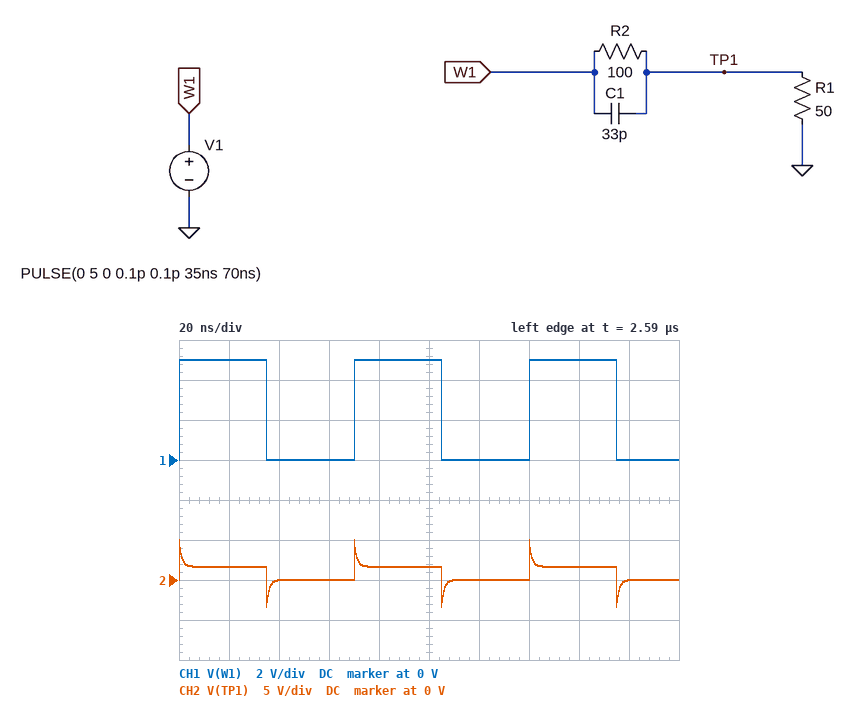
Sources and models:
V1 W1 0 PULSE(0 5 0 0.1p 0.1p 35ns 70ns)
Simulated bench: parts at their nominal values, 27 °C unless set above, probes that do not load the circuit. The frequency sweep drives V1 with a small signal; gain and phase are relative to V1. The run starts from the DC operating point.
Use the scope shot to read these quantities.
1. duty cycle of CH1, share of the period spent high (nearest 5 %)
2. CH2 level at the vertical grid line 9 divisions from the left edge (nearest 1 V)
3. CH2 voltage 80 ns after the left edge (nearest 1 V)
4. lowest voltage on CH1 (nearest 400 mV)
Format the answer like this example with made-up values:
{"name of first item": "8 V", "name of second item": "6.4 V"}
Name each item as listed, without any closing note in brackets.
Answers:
{"duty cycle of CH1, share of the period spent high": "50 %", "CH2 level at the vertical grid line 9 divisions from the left edge": "0 V", "CH2 voltage 80 ns after the left edge": "2 V", "lowest voltage on CH1": "0 V"}
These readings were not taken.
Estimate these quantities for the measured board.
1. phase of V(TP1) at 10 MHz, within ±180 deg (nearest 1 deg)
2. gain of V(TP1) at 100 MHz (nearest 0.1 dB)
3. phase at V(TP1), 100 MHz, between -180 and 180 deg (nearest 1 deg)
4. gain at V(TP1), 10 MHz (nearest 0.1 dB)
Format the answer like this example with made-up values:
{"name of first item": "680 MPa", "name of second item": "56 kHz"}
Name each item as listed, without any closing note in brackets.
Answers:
{"phase of V(TP1) at 10 MHz, within ±180 deg": "8 deg", "gain of V(TP1) at 100 MHz": "-4.0 dB", "phase at V(TP1), 100 MHz, between -180 and 180 deg": "30 deg", "gain at V(TP1), 10 MHz": "-9.4 dB"}
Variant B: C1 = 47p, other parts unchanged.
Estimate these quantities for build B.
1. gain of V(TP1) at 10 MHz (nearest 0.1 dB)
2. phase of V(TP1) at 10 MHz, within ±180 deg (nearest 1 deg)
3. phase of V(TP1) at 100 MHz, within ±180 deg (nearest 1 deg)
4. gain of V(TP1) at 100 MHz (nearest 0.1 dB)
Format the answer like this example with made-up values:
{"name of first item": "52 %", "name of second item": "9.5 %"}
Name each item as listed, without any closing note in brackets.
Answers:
{"gain of V(TP1) at 10 MHz": "-9.2 dB", "phase of V(TP1) at 10 MHz, within ±180 deg": "11 deg", "phase of V(TP1) at 100 MHz, within ±180 deg": "27 deg", "gain of V(TP1) at 100 MHz": "-2.6 dB"}
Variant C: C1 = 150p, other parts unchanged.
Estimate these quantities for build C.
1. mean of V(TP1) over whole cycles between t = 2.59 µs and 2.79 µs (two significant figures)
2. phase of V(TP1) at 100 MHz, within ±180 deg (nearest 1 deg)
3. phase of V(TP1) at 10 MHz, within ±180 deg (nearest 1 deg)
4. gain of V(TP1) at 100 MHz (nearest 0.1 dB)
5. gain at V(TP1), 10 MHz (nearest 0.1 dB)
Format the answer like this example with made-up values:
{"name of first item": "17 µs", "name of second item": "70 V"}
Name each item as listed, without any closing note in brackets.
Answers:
{"mean of V(TP1) over whole cycles between t = 2.59 µs and 2.79 µs": "830 mV", "phase of V(TP1) at 100 MHz, within ±180 deg": "12 deg", "phase of V(TP1) at 10 MHz, within ±180 deg": "26 deg", "gain of V(TP1) at 100 MHz": "-0.4 dB", "gain at V(TP1), 10 MHz": "-7.2 dB"}
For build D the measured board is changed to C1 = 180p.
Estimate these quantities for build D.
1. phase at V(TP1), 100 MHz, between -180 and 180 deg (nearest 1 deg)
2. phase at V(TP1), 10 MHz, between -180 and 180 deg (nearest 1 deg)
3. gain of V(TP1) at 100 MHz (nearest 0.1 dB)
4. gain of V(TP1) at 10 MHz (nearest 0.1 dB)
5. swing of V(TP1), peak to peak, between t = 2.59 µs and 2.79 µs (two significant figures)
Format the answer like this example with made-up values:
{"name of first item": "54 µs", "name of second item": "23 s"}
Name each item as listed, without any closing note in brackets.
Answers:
{"phase at V(TP1), 100 MHz, between -180 and 180 deg": "10 deg", "phase at V(TP1), 10 MHz, between -180 and 180 deg": "28 deg", "gain of V(TP1) at 100 MHz": "-0.3 dB", "gain of V(TP1) at 10 MHz": "-6.5 dB", "swing of V(TP1), peak to peak, between t = 2.59 µs and 2.79 µs": "8.3 V"}
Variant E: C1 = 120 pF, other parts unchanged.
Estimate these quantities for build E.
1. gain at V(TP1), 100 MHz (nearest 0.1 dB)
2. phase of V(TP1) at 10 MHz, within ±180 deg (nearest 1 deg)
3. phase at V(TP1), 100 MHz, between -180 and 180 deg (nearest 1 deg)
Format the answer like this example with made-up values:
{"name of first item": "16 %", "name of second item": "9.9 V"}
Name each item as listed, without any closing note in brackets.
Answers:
{"gain at V(TP1), 100 MHz": "-0.6 dB", "phase of V(TP1) at 10 MHz, within ±180 deg": "23 deg", "phase at V(TP1), 100 MHz, between -180 and 180 deg": "14 deg"}
